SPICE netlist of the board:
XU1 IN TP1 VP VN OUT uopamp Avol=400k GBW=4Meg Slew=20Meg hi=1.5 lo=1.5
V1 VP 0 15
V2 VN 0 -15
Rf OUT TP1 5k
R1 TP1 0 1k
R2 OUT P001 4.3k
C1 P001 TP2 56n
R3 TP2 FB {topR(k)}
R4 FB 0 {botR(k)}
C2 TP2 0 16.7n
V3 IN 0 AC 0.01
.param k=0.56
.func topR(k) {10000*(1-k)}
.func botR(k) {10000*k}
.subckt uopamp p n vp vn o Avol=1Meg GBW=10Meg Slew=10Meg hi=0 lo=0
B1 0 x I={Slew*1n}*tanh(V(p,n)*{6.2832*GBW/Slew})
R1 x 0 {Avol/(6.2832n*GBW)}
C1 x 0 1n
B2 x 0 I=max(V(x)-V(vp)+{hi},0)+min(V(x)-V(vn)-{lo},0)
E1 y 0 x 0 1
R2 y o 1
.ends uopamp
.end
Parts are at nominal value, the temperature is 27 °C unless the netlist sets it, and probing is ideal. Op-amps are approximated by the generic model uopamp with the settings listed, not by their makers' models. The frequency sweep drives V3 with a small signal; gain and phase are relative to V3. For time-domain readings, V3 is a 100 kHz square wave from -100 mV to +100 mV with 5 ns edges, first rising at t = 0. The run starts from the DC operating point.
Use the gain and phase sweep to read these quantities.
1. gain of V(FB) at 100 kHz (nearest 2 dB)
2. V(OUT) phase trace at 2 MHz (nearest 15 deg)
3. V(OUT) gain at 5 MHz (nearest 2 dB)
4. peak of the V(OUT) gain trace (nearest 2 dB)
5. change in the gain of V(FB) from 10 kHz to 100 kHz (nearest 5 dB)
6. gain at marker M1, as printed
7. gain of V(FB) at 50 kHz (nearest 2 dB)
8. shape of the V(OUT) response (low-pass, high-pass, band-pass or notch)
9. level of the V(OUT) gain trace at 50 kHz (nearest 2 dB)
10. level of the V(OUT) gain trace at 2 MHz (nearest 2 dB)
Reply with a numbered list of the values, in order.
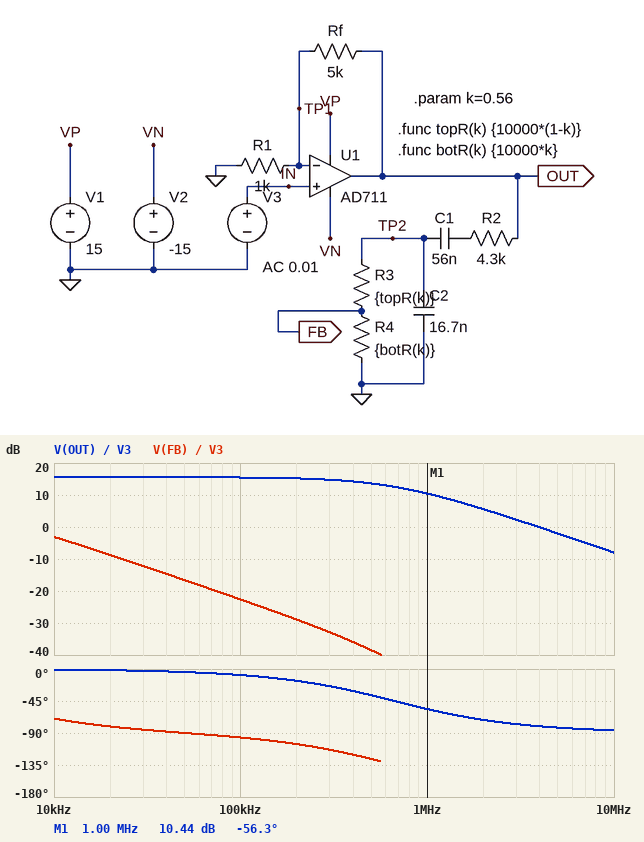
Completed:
1. -22 dB
2. -75 deg
3. -2 dB
4. 16 dB
5. -20 dB
6. 10.44 dB
7. -16 dB
8. low-pass
9. 16 dB
10. 6 dB
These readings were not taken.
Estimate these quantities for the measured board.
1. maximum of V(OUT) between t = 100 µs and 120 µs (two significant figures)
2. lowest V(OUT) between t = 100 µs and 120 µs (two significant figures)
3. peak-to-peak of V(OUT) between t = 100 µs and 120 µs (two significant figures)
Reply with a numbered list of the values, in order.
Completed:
1. 600 mV
2. -600 mV
3. 1.2 V
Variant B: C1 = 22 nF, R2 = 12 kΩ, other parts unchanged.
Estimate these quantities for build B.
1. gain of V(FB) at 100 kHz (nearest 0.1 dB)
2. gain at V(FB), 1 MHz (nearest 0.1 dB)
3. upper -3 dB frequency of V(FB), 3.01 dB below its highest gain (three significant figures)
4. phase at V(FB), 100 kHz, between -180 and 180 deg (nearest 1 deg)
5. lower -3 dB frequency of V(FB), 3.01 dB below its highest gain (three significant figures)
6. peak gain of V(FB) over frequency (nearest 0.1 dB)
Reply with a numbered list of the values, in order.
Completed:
1. -31.6 dB
2. -56.6 dB
3. 2.57 kHz
4. -97 deg
5. 223 Hz
6. 1.1 dB
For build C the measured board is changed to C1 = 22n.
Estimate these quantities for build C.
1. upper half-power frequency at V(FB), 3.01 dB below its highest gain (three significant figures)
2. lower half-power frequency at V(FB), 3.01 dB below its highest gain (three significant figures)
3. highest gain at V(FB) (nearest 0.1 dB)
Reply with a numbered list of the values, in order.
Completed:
1. 5.16 kHz
2. 311 Hz
3. 3.7 dB
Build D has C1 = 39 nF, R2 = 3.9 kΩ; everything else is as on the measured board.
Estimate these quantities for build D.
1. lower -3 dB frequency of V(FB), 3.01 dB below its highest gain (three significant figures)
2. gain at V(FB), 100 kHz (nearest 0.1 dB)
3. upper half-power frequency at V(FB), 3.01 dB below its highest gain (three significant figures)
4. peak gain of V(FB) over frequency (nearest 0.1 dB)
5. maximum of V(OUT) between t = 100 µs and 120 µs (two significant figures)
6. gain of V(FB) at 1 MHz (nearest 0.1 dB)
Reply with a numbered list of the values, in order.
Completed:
1. 214 Hz
2. -21.8 dB
3. 4.66 kHz
4. 5.3 dB
5. 600 mV
6. -46.8 dB
